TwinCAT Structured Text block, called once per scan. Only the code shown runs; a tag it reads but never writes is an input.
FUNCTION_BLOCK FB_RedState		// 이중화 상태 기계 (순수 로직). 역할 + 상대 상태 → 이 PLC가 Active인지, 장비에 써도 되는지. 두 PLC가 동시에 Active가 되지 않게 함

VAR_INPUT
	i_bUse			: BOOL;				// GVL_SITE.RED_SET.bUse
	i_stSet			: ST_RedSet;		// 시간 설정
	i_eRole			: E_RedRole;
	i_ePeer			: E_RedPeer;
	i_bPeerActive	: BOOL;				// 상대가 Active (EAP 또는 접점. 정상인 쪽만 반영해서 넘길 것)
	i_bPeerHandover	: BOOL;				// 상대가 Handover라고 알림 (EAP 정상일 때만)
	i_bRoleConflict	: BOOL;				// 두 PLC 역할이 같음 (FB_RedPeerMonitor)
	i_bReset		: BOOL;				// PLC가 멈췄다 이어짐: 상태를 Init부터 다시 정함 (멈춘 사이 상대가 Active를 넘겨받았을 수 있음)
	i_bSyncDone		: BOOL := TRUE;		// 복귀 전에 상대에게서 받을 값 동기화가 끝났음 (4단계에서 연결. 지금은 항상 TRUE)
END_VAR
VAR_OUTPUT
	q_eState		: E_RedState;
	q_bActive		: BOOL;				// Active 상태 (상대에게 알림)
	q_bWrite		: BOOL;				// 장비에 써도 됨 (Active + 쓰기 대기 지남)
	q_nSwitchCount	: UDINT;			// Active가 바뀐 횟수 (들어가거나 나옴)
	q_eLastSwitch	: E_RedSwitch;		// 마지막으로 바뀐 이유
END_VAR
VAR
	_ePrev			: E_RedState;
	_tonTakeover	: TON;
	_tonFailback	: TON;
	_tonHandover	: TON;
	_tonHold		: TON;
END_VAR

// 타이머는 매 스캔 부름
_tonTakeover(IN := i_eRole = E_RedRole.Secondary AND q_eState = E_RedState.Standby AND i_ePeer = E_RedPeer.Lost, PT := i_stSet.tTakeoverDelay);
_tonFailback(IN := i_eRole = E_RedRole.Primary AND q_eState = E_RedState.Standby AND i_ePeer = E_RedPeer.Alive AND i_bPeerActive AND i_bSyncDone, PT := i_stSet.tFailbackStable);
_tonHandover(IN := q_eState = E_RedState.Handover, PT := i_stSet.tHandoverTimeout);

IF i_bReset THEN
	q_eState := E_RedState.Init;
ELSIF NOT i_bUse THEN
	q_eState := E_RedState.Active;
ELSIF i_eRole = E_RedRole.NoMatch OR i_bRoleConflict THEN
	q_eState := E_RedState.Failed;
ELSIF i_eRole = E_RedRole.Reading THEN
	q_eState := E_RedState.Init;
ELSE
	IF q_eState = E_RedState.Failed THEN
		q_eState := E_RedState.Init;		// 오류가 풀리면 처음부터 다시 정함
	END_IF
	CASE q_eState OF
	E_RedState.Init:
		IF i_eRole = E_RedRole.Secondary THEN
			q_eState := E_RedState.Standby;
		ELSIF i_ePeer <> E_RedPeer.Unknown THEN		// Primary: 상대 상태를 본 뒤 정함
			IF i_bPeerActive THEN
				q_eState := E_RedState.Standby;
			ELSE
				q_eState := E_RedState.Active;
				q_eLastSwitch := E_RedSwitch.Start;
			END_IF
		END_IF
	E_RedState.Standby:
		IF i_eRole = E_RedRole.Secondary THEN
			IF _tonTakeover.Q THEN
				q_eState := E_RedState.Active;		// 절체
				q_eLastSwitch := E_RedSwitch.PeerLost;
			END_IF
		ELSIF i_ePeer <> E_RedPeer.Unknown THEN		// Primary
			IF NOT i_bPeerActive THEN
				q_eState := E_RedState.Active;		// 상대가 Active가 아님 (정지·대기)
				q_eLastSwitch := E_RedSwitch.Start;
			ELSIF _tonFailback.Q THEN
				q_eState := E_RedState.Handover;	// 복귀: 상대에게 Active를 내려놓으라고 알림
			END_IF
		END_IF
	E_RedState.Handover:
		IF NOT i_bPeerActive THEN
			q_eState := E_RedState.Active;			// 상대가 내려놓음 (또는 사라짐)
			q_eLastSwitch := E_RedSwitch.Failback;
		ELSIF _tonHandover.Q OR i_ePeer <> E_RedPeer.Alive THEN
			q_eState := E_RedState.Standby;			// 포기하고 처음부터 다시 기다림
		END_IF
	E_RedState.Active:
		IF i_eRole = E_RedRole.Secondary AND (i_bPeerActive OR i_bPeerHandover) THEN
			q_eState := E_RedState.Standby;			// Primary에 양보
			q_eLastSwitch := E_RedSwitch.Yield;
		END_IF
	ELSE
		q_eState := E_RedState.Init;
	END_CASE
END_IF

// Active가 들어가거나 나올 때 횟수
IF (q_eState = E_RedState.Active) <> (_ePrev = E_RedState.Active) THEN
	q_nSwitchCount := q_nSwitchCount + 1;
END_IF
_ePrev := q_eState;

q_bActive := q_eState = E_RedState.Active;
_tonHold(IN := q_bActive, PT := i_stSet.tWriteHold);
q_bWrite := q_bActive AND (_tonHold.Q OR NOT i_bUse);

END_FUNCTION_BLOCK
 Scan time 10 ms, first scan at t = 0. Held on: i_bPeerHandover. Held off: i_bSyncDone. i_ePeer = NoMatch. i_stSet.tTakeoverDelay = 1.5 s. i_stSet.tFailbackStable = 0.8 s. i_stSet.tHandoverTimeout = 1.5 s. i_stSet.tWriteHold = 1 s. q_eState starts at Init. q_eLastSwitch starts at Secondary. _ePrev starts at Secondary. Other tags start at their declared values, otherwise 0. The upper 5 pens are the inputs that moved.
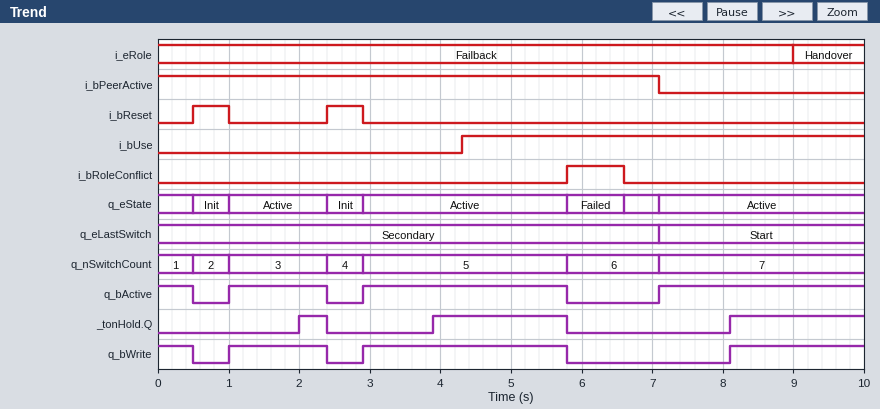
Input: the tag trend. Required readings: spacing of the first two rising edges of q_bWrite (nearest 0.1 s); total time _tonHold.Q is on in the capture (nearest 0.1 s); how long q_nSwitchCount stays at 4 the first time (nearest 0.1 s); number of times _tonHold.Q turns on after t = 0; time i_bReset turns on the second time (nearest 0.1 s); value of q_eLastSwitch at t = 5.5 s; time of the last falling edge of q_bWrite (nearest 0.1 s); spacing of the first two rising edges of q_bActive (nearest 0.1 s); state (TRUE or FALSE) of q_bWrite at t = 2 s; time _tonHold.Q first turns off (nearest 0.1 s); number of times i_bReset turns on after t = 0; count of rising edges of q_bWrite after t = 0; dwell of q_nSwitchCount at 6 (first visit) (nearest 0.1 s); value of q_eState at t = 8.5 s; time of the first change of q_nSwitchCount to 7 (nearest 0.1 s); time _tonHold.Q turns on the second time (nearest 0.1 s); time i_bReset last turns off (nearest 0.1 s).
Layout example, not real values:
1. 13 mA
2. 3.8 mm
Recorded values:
1. 1.9 s
2. 4.2 s
3. 0.5 s
4. 3
5. 2.4 s
6. Secondary
7. 5.8 s
8. 1.9 s
9. TRUE
10. 2.4 s
11. 2
12. 3
13. 1.3 s
14. Active
15. 7.1 s
16. 3.9 s
17. 2.9 s
